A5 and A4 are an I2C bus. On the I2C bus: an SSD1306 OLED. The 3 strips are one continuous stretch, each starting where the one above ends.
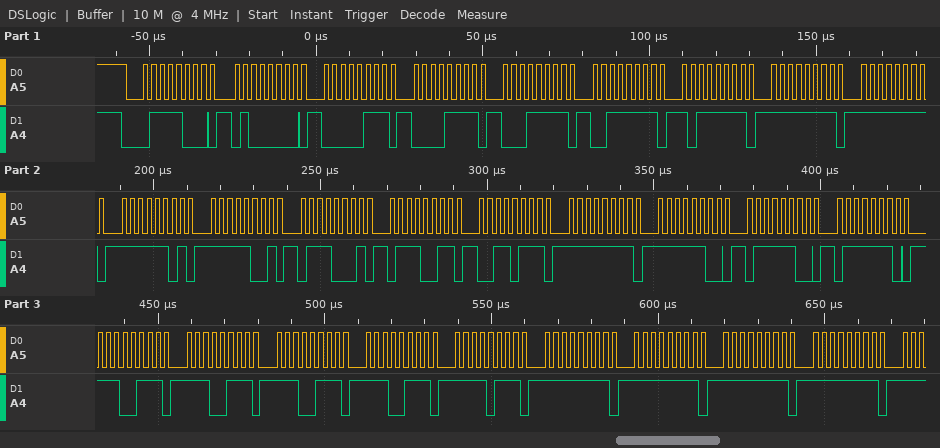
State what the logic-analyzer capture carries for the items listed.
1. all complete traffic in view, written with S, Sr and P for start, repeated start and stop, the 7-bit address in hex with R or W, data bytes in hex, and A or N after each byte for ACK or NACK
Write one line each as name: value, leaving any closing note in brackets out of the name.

all complete traffic in view, written with S, Sr and P for start, repeated start and stop, the 7-bit address in hex with R or W, data bytes in hex, and A or N after each byte for ACK or NACK: S 3CW A 40 A 07 A 0F A 1F A 3F A BF A FF A FF A FD A F9 A 71 A 73 A 37 A FF A FC A 7C A 7E A E7 A E7 A E7 A E7 A F7 A FF A FF A FF A FF A
